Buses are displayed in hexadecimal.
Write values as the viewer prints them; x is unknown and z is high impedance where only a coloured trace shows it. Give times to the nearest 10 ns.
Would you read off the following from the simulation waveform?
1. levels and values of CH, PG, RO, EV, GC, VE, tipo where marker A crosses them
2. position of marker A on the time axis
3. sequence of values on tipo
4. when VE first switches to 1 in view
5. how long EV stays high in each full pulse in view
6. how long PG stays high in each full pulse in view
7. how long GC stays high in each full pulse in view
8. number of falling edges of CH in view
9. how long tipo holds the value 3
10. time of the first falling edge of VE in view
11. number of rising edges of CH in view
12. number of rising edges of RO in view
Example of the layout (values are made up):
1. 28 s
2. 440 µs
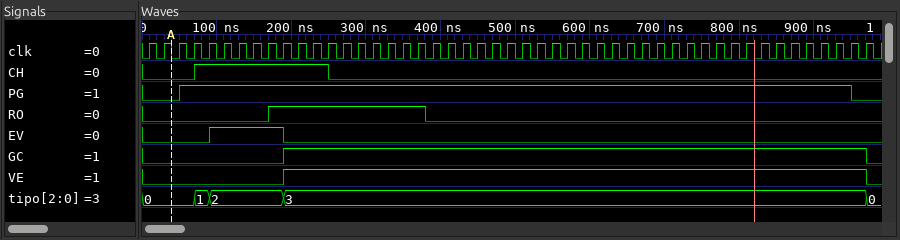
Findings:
1. CH=0, PG=0, RO=0, EV=0, GC=0, VE=0, tipo=0
2. 40 ns
3. 0, 1, 2, 3, 0
4. 190 ns
5. 100 ns
6. 900 ns
7. 780 ns
8. 1
9. 780 ns
10. 970 ns
11. 1
12. 1
